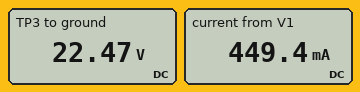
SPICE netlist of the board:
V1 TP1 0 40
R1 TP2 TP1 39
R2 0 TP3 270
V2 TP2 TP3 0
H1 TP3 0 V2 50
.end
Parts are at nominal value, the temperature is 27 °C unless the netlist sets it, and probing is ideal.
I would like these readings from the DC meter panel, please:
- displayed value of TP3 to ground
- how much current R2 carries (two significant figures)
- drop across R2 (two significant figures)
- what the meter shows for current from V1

22.47 V
83 mA
22 V
449.4 mA
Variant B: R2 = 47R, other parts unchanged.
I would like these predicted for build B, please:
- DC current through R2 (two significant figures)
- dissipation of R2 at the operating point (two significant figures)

480 mA
11 W
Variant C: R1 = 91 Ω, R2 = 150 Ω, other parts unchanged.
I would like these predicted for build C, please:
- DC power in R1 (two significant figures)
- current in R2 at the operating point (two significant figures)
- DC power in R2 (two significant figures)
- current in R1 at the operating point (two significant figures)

7.3 W
95 mA
1.3 W
280 mA
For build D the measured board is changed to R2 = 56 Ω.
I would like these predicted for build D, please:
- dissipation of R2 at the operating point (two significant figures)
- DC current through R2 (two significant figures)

9.0 W
400 mA
